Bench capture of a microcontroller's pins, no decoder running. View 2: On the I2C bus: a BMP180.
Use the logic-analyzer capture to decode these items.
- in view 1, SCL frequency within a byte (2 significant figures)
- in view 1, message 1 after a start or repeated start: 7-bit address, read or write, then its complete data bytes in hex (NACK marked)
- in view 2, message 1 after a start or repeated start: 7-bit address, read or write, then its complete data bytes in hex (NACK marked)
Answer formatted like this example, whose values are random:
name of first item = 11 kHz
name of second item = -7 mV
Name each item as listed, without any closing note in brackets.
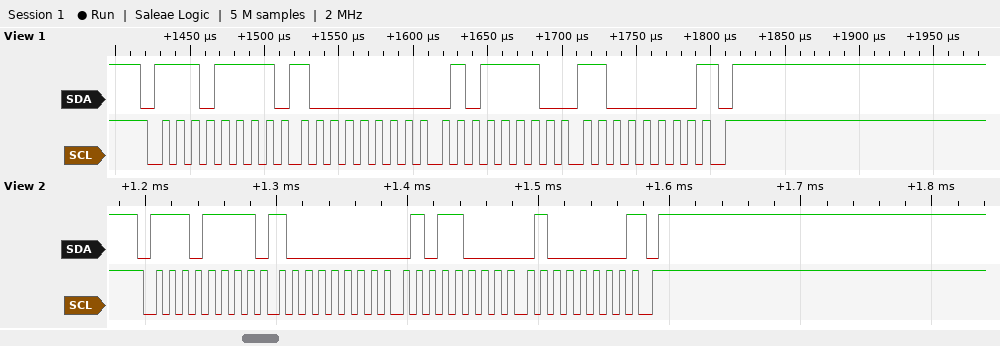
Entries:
in view 1, SCL frequency within a byte = 100 kHz
in view 1, message 1 after a start or repeated start: 7-bit address, read or write, then its complete data bytes in hex = 0x77 read: 80 5E C0 NACK
in view 2, message 1 after a start or repeated start: 7-bit address, read or write, then its complete data bytes in hex = 0x77 read: 80 58 40 NACK
